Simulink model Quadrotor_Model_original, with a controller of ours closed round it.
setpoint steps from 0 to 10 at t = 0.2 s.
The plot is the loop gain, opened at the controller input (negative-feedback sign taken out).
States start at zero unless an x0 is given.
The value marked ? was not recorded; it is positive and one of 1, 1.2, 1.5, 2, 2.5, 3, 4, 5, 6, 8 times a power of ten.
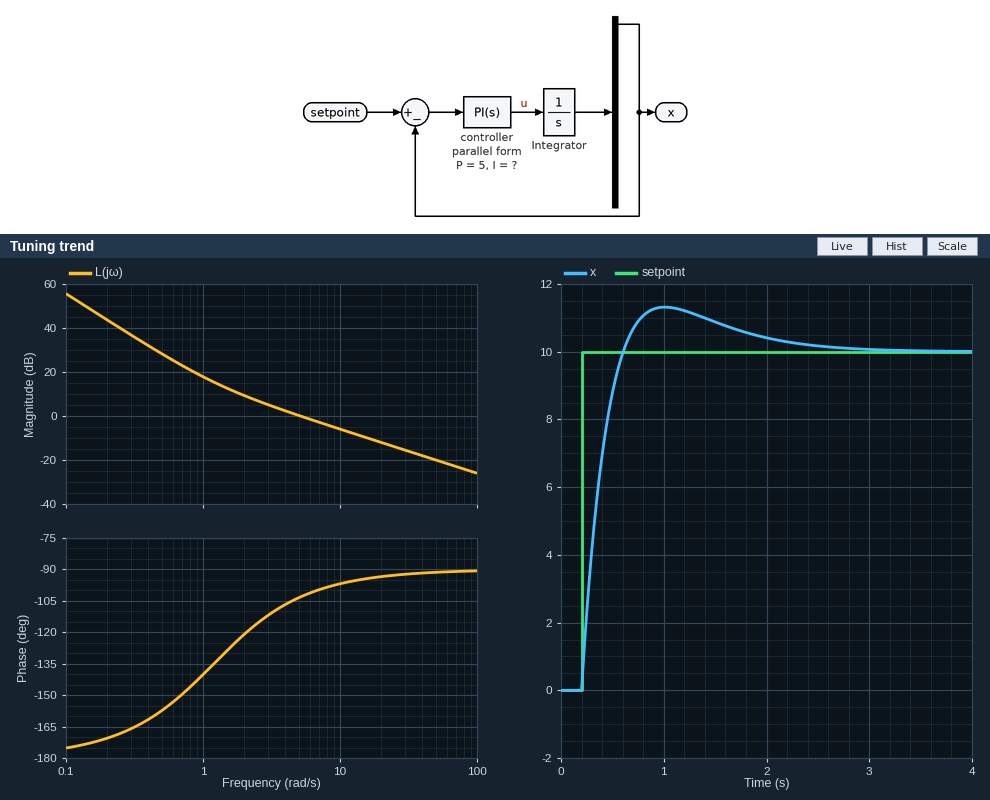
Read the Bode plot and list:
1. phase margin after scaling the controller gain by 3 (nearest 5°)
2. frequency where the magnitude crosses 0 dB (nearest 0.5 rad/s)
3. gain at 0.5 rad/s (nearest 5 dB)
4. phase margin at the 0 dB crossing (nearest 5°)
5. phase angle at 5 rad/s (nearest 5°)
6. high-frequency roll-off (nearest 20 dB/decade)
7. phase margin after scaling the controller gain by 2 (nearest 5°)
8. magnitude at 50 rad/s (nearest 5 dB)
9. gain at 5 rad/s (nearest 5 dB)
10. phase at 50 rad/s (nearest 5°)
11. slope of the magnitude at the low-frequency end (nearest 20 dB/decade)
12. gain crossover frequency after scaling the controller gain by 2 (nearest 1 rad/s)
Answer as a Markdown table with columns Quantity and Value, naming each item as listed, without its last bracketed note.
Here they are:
| Quantity | Value |
|---|---|
| phase margin after scaling the controller gain by 3 | 85° |
| frequency where the magnitude crosses 0 dB | 5.0 rad/s |
| gain at 0.5 rad/s | 30 dB |
| phase margin at the 0 dB crossing | 75° |
| phase angle at 5 rad/s | -105° |
| high-frequency roll-off | -20 dB/decade |
| phase margin after scaling the controller gain by 2 | 85° |
| magnitude at 50 rad/s | -20 dB |
| gain at 5 rad/s | 0 dB |
| phase at 50 rad/s | -90° |
| slope of the magnitude at the low-frequency end | -40 dB/decade |
| gain crossover frequency after scaling the controller gain by 2 | 10 rad/s |
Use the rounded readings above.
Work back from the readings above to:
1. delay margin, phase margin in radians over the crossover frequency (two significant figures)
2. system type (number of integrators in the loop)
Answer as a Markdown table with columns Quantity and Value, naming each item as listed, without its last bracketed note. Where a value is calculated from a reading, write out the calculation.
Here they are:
| Quantity | Value |
|---|---|
| delay margin, phase margin in radians over the crossover frequency | 75 × π / 180 / 5 = 0.26 s |
| system type | 2 |
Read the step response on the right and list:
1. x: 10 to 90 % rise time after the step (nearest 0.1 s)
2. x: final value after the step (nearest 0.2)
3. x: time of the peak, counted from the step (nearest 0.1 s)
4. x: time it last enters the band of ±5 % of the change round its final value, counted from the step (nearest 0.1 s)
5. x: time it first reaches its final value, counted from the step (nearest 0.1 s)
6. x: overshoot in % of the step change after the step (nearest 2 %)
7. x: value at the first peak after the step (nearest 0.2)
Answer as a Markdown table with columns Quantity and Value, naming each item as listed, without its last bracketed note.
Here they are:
| Quantity | Value |
|---|---|
| x: 10 to 90 % rise time after the step | 0.3 s |
| x: final value after the step | 10.0 |
| x: time of the peak, counted from the step | 0.8 s |
| x: time it last enters the band of ±5 % of the change round its final value, counted from the step | 1.7 s |
| x: time it first reaches its final value, counted from the step | 0.4 s |
| x: overshoot in % of the step change after the step | 14 % |
| x: value at the first peak after the step | 11.4 |
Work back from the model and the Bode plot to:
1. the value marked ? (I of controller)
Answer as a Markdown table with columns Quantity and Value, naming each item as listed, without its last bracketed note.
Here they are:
| Quantity | Value |
|---|---|
| the value marked ? | 6 |
